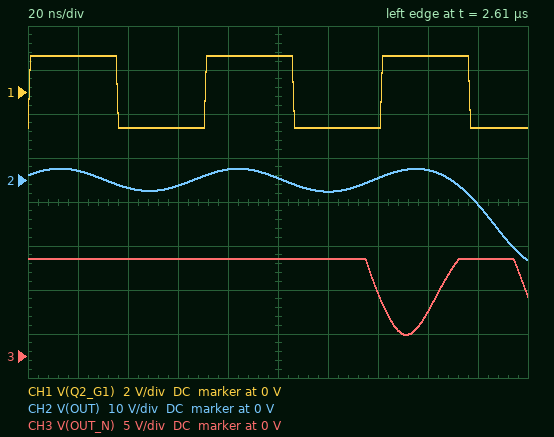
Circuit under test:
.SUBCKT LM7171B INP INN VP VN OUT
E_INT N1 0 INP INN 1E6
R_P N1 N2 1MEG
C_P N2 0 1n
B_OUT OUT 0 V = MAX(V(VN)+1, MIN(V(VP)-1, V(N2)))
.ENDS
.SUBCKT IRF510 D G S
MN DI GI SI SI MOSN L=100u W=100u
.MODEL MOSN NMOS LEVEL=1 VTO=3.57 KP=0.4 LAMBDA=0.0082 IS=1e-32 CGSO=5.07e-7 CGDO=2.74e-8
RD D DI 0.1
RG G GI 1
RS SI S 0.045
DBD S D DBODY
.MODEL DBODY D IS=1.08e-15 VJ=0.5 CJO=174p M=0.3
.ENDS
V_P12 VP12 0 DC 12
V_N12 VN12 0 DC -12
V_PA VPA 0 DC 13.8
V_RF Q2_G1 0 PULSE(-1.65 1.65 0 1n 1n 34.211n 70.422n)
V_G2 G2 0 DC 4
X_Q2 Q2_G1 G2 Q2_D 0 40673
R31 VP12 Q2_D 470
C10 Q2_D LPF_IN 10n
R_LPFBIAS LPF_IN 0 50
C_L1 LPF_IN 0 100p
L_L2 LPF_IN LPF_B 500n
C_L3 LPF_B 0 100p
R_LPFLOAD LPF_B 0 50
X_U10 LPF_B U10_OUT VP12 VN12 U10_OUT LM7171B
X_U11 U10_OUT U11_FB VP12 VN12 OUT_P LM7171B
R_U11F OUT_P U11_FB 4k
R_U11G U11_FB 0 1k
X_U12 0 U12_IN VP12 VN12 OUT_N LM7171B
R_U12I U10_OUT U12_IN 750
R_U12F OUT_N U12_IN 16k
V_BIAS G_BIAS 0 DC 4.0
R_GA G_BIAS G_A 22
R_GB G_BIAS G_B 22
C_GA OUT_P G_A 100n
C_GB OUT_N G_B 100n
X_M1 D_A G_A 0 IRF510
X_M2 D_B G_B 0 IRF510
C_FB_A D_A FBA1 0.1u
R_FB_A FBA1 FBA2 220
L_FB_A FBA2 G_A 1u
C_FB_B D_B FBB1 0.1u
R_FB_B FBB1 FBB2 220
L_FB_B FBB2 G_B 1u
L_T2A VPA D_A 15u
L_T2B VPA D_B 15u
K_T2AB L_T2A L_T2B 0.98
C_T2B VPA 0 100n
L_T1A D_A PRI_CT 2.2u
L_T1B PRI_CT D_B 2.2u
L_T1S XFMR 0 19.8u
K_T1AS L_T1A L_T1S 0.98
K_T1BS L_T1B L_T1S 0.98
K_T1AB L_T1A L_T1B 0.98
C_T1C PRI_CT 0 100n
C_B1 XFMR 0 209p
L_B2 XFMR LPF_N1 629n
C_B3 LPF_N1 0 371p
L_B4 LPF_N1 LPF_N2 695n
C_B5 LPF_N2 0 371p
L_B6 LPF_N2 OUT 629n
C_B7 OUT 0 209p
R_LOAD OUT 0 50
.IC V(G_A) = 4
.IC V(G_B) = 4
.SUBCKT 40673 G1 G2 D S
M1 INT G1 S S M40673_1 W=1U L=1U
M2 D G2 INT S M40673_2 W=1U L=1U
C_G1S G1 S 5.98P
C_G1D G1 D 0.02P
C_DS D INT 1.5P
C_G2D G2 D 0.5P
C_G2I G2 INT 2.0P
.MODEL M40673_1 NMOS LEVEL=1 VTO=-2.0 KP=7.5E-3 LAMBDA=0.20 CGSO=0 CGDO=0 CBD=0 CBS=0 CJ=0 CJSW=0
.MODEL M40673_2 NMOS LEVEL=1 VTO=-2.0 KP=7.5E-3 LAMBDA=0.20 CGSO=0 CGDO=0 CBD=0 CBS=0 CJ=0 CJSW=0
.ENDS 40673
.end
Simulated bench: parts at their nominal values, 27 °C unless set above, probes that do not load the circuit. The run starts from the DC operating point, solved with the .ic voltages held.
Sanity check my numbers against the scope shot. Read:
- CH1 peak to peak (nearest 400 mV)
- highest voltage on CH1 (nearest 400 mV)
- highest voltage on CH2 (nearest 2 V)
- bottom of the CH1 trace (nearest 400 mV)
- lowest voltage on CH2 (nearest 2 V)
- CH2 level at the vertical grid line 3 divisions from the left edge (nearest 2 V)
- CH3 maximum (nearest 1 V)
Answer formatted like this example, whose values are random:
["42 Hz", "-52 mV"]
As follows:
["3.2 V", "1.6 V", "2 V", "-1.6 V", "-18 V", "-2 V", "11 V"]
